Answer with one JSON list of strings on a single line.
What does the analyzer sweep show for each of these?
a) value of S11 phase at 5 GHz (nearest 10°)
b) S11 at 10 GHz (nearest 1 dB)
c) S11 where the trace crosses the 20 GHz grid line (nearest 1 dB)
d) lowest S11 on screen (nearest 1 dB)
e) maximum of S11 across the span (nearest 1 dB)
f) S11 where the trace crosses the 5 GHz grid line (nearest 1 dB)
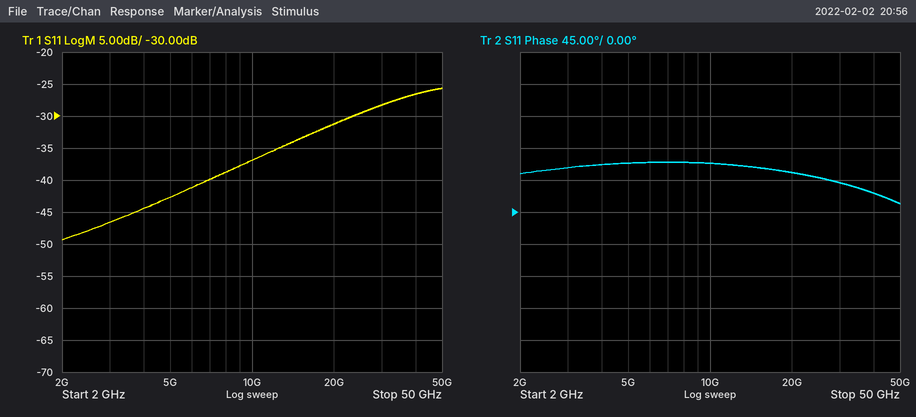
["70°", "-37 dB", "-31 dB", "-49 dB", "-26 dB", "-43 dB"]
